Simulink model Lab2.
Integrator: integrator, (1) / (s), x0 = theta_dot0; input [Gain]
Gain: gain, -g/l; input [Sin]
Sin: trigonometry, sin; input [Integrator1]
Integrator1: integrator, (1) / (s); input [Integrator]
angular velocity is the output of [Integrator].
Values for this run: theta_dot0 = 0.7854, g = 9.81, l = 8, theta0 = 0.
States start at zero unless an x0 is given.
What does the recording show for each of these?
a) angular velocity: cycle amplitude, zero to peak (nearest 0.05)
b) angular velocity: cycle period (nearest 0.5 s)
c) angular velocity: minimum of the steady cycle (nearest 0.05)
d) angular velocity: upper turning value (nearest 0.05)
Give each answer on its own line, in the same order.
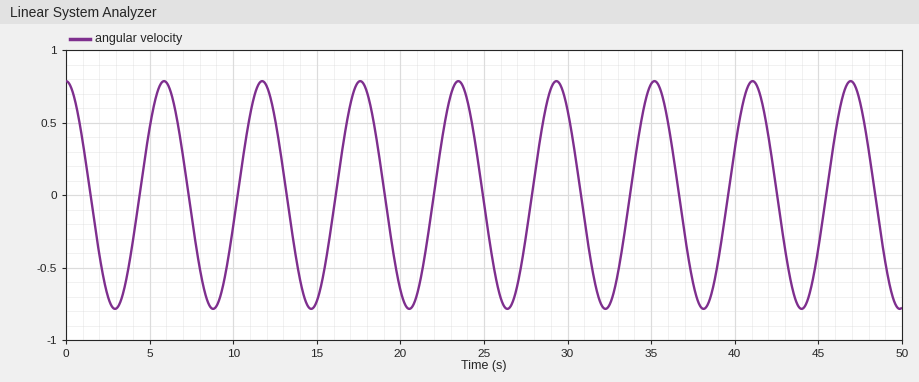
0.80
6.0 s
-0.80
0.80
